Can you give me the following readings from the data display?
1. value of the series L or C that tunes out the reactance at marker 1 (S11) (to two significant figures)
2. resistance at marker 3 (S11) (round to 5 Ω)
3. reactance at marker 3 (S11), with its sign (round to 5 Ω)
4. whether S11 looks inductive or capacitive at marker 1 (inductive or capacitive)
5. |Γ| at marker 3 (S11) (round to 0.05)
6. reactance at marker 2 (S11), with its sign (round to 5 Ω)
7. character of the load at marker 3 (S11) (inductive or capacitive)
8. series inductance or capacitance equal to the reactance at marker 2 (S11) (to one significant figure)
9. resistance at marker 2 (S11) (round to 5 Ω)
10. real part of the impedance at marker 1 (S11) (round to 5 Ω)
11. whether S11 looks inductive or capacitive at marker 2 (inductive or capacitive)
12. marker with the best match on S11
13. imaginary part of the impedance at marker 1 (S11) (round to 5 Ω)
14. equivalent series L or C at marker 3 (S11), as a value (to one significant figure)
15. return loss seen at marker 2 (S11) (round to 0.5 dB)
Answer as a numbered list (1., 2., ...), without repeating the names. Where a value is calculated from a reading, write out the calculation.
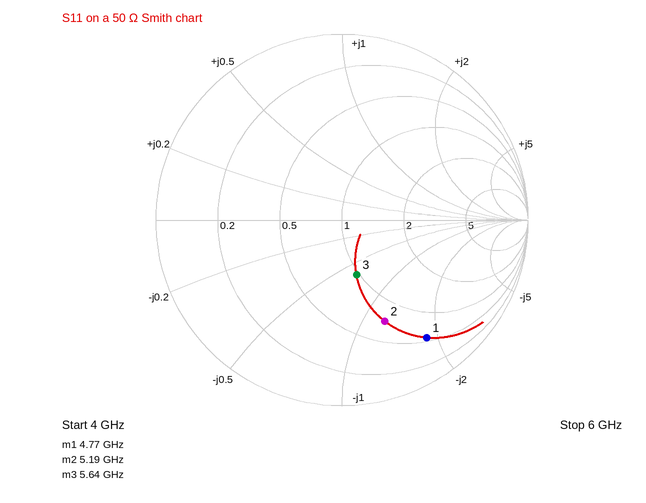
1. L = 90 Ω/(2π × 4.77 GHz) ≈ 3.0 nH
2. 50 Ω
3. -30 Ω
4. capacitive
5. 0.30
6. -60 Ω
7. capacitive
8. C = 1/(2π × 5.19 GHz × 60 Ω) ≈ 511 fF, so 500 fF to one significant figure
9. 35 Ω
10. 30 Ω
11. capacitive
12. marker 3
13. -90 Ω
14. C = 1/(2π × 5.64 GHz × 30 Ω) ≈ 941 fF, so 900 fF to one significant figure
15. 4.5 dB
